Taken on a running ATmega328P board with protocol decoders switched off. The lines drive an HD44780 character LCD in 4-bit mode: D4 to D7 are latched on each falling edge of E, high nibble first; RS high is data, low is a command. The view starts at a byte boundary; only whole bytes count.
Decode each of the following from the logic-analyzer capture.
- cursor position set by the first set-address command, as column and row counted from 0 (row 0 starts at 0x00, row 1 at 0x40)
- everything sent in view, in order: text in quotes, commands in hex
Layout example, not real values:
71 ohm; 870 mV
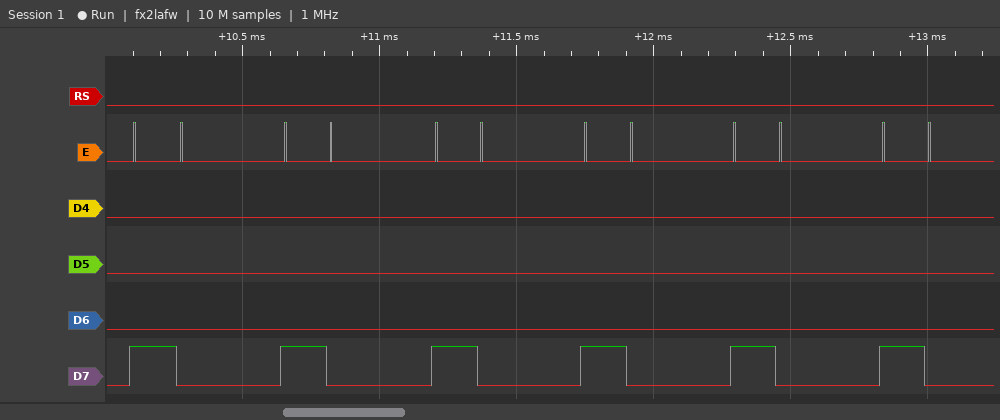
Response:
column 0, row 0; 0x80 0x80 0x80 0x80 0x80 0x80
